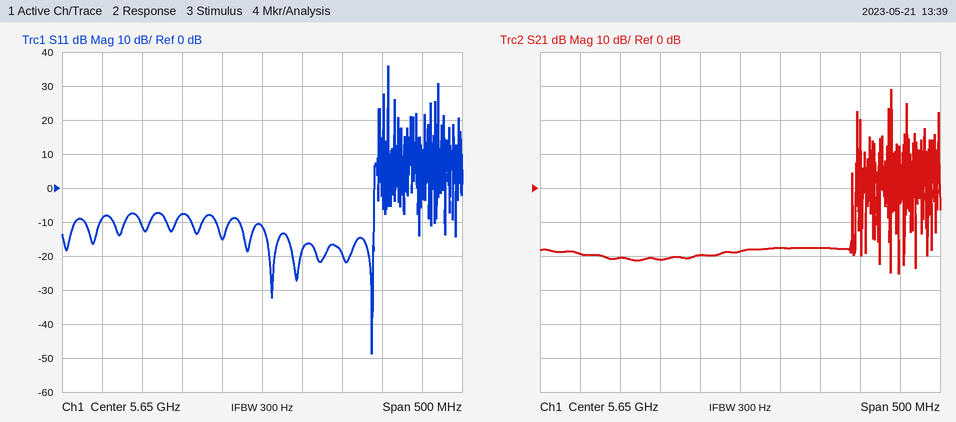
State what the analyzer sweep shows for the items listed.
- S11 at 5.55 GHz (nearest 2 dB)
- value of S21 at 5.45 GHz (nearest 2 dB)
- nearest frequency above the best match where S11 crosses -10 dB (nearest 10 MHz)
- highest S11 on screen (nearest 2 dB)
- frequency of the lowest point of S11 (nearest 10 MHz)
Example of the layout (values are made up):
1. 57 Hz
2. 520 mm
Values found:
1. -8 dB
2. -20 dB
3. 5.79 GHz
4. 36 dB
5. 5.79 GHz
